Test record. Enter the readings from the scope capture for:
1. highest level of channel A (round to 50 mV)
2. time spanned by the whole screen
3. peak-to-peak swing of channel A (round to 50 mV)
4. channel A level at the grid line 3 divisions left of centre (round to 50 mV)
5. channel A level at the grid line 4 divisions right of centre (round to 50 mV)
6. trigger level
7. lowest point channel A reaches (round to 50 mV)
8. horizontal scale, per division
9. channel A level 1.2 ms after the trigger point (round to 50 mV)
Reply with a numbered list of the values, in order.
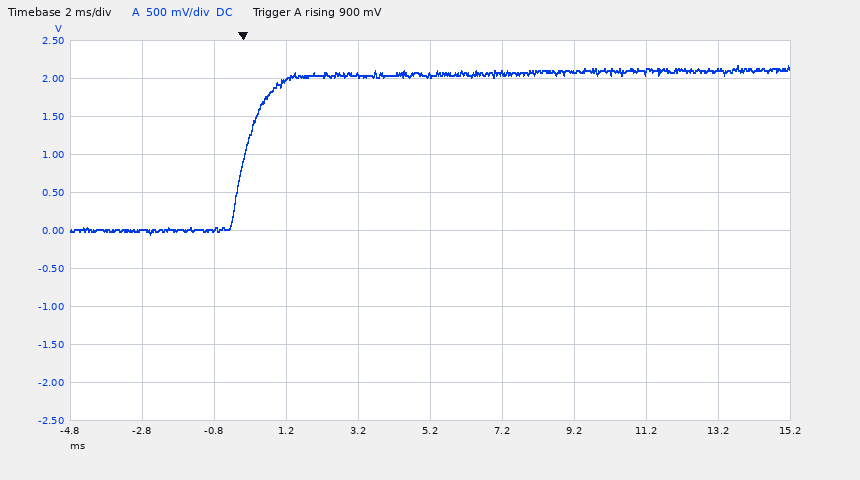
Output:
1. 2.15 V
2. 20 ms
3. 2.20 V
4. 0 mV
5. 2.10 V
6. 900 mV
7. -50 mV
8. 2 ms
9. 2.00 V
